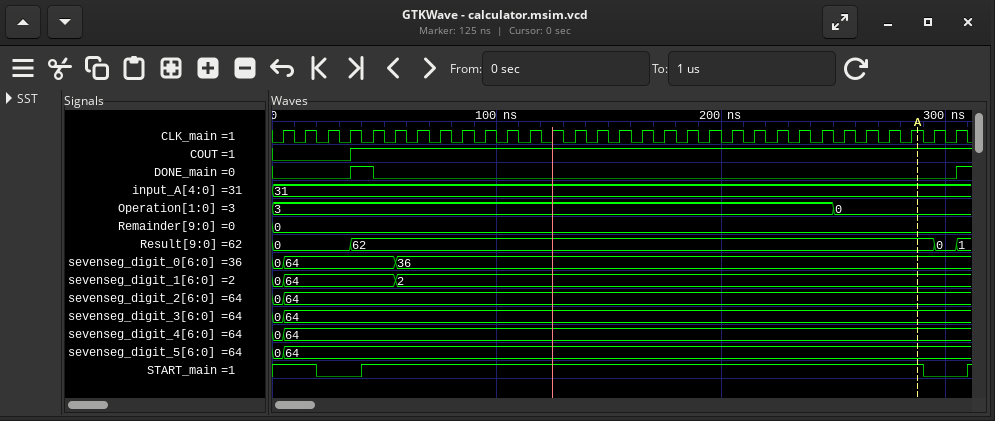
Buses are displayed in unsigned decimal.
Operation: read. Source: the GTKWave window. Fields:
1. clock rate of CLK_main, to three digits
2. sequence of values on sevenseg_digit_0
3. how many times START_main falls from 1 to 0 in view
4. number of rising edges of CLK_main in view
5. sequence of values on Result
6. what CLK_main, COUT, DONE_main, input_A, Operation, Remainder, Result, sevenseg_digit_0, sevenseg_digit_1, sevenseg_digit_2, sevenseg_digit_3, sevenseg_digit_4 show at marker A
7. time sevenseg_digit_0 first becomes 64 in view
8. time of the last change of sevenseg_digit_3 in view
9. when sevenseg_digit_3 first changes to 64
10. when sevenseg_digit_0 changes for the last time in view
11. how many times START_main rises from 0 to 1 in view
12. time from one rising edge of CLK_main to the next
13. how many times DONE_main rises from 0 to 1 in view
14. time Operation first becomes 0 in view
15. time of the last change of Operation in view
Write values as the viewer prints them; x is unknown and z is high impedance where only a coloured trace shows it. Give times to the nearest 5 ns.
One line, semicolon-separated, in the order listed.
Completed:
100 MHz; 0, 64, 36; 2; 31; 0, 62, 0, 1; CLK_main=1, COUT=1, DONE_main=0, input_A=31, Operation=0, Remainder=0, Result=62, sevenseg_digit_0=36, sevenseg_digit_1=2, sevenseg_digit_2=64, sevenseg_digit_3=64, sevenseg_digit_4=64; 5 ns; 5 ns; 5 ns; 55 ns; 2; 10 ns; 2; 250 ns; 250 ns
